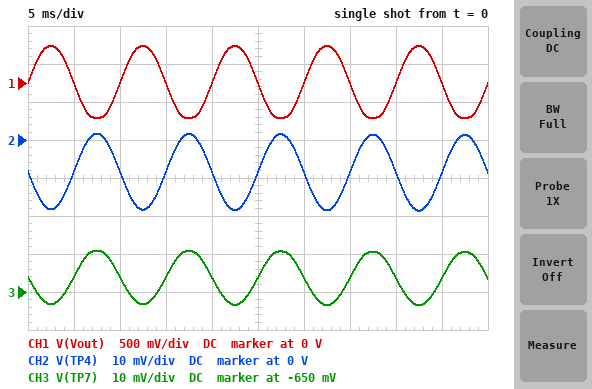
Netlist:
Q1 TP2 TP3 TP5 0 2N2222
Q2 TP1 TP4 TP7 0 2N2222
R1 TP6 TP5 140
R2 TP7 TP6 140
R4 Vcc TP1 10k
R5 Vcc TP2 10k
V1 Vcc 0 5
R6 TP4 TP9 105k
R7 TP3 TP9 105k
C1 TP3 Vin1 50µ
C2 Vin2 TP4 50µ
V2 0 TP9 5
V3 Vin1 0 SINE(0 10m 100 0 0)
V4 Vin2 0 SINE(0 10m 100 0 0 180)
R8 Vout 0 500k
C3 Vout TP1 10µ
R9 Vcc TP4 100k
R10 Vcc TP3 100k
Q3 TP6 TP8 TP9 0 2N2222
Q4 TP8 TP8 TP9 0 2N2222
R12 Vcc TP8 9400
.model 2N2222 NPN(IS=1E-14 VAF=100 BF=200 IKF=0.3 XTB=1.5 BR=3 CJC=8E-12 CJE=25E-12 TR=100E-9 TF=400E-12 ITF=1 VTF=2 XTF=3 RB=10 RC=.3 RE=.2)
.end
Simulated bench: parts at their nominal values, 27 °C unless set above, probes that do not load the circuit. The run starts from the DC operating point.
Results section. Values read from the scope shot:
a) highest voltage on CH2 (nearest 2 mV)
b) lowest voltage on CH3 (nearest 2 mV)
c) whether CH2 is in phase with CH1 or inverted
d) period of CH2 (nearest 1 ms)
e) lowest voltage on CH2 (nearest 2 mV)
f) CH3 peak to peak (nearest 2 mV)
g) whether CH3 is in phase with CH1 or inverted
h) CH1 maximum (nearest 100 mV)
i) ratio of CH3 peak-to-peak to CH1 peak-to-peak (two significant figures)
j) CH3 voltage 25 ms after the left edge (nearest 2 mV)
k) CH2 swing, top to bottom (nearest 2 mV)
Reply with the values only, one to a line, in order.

2 mV
-654 mV
inverted
10 ms
-18 mV
14 mV
inverted
500 mV
0.015
-646 mV
20 mV
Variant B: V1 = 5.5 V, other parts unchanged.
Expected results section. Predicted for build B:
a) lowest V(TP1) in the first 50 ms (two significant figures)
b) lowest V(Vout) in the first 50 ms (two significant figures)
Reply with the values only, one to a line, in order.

-300 mV
-440 mV
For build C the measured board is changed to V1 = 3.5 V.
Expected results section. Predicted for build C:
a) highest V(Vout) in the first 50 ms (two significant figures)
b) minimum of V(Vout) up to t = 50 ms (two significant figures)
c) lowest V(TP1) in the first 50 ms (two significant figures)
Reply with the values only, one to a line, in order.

480 mV
-480 mV
-1.2 V
